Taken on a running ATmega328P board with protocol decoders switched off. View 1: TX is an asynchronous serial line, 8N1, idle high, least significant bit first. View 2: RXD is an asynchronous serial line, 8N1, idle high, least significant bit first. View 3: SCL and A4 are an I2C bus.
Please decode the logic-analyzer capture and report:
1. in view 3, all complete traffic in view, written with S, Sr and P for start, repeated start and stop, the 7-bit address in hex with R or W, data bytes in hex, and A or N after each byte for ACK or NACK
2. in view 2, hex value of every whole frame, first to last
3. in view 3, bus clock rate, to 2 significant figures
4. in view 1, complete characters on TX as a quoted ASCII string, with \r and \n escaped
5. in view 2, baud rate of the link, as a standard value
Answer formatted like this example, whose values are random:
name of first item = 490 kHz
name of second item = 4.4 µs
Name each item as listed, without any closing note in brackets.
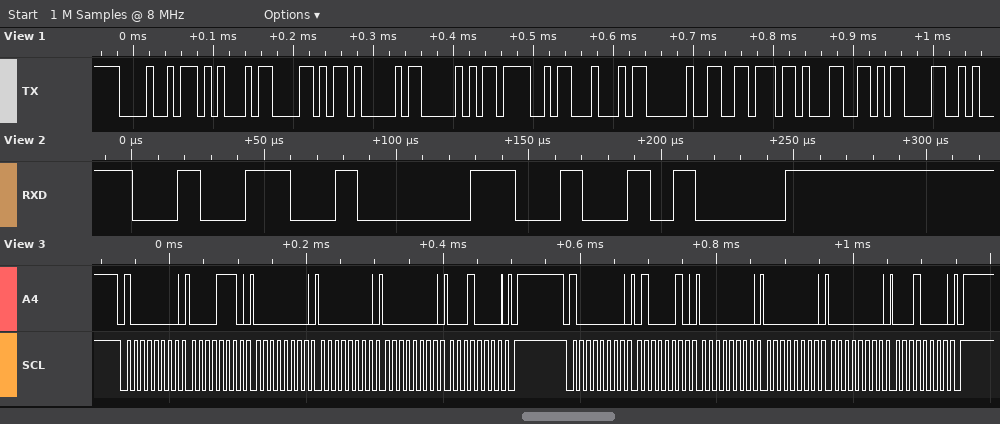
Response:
in view 3, all complete traffic in view, written with S, Sr and P for start, repeated start and stop, the 7-bit address in hex with R or W, data bytes in hex, and A or N after each byte for ACK or NACK = S 40W A 0E A 00 A 00 A 00 A 10 A P S 40W A 42 A 00 A 00 A 00 A 10 A P
in view 2, hex value of every whole frame, first to last = 32 30 0A
in view 3, bus clock rate, to 2 significant figures = 100 kHz
in view 1, complete characters on TX as a quoted ASCII string, with \r and \n escaped = "HEXAPOD v1\r"
in view 2, baud rate of the link, as a standard value = 115200 baud
